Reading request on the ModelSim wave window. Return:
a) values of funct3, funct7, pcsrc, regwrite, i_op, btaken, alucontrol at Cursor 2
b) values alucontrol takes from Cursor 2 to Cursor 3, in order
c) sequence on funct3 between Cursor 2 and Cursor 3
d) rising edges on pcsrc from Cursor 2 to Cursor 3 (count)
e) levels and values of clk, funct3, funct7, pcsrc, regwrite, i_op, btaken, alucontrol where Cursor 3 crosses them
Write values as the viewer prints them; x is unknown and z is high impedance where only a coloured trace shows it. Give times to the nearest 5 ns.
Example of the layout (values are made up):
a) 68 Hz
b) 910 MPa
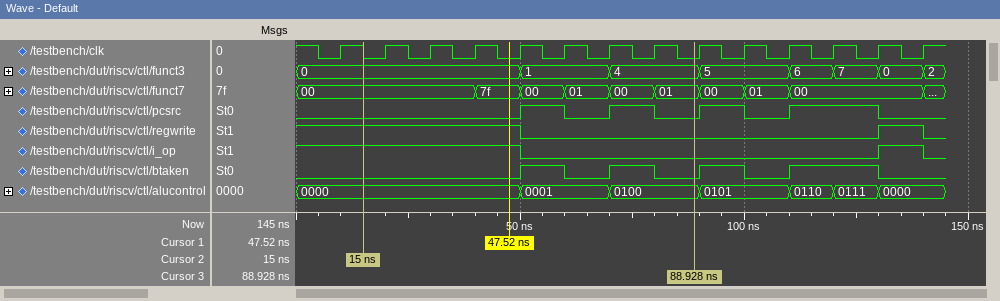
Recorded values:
a) funct3=0, funct7=00, pcsrc=0, regwrite=1, i_op=1, btaken=0, alucontrol=0000
b) 0000, 0001, 0100
c) 0, 1, 4
d) 2
e) clk=0, funct3=4, funct7=01, pcsrc=0, regwrite=0, i_op=0, btaken=0, alucontrol=0100
